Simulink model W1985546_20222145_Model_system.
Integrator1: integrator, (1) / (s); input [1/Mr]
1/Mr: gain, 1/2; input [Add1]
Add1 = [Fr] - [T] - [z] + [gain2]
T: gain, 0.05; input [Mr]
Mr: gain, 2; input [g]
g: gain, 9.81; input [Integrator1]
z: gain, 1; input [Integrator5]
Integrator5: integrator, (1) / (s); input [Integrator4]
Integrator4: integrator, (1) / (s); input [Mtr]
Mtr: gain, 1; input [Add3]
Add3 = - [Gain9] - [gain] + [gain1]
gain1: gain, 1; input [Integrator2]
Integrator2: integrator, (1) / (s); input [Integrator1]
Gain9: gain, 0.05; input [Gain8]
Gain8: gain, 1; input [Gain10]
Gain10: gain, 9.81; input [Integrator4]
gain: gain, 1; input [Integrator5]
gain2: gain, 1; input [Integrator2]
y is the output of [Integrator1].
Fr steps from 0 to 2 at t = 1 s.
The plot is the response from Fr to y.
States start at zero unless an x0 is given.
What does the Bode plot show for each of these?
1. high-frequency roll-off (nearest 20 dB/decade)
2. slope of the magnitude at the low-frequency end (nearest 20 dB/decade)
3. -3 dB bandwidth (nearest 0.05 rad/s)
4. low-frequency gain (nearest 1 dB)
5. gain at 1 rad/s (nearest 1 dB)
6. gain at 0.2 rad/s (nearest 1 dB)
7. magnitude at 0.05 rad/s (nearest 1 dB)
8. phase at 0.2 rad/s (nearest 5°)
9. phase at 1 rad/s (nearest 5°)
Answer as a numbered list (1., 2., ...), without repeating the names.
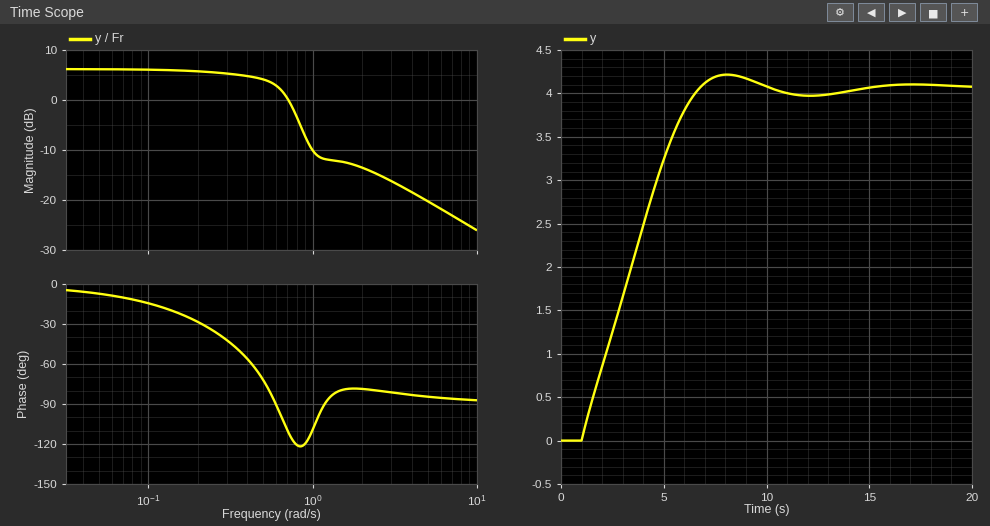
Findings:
1. -20 dB/decade
2. 0 dB/decade
3. 0.60 rad/s
4. 6 dB
5. -10 dB
6. 6 dB
7. 6 dB
8. -30°
9. -110°
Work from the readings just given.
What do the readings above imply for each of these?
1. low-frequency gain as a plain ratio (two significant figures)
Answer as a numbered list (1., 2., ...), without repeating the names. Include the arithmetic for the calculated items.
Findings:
1. 10^(6 / 20) = 2.0
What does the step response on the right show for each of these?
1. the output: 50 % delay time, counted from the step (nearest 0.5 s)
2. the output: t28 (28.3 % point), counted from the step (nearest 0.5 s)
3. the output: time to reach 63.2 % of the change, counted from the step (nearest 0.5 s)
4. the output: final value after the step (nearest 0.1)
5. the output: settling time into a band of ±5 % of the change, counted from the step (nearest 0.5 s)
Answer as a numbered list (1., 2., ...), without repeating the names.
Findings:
1. 2.5 s
2. 1.5 s
3. 3.0 s
4. 4.1
5. 5.0 s
